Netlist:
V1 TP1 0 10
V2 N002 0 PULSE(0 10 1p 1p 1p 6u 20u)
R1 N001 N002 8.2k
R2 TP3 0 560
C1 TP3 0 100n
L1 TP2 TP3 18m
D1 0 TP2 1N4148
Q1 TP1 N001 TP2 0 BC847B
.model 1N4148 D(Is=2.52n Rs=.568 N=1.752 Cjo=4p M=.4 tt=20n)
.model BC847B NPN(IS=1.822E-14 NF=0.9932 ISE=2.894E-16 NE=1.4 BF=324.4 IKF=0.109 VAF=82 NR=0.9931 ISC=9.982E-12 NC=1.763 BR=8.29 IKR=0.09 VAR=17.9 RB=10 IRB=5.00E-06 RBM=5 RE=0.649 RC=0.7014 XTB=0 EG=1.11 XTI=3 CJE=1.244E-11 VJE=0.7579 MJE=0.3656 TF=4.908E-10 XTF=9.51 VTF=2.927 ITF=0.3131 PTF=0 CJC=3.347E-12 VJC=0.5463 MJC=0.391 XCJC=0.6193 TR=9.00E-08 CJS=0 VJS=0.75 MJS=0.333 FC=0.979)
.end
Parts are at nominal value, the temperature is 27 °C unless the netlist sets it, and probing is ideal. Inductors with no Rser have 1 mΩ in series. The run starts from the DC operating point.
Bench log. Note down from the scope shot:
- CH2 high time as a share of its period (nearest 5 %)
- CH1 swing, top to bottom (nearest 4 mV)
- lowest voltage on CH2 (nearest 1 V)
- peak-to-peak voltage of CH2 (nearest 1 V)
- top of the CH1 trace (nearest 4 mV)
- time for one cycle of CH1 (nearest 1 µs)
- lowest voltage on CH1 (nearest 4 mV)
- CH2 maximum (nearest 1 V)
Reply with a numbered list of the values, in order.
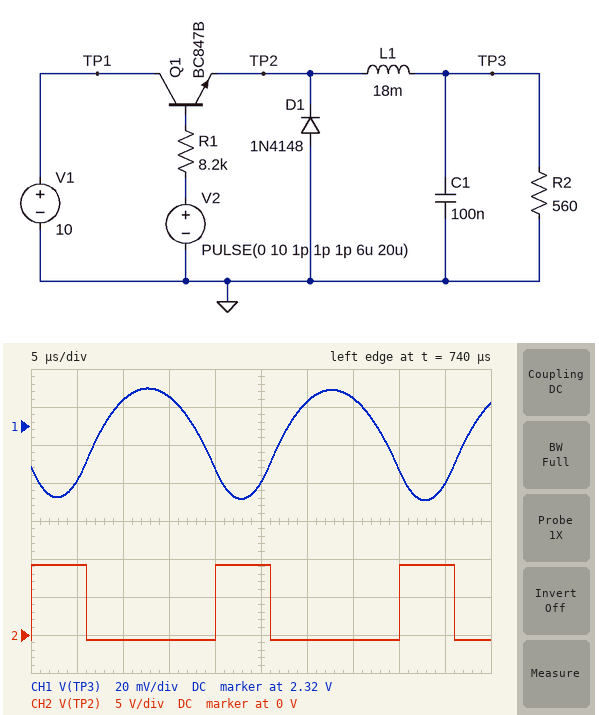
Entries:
1. 30 %
2. 60 mV
3. -1 V
4. 10 V
5. 2.340 V
6. 20 µs
7. 2.280 V
8. 9 V
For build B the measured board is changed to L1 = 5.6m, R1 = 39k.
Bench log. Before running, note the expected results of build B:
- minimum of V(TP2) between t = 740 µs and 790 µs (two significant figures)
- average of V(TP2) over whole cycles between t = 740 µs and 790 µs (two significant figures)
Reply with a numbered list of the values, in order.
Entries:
1. -670 mV
2. 2.2 V
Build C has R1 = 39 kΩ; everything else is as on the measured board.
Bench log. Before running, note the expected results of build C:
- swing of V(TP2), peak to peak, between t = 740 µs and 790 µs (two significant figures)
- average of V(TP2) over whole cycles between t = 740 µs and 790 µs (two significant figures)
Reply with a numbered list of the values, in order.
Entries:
1. 9.6 V
2. 2.2 V
